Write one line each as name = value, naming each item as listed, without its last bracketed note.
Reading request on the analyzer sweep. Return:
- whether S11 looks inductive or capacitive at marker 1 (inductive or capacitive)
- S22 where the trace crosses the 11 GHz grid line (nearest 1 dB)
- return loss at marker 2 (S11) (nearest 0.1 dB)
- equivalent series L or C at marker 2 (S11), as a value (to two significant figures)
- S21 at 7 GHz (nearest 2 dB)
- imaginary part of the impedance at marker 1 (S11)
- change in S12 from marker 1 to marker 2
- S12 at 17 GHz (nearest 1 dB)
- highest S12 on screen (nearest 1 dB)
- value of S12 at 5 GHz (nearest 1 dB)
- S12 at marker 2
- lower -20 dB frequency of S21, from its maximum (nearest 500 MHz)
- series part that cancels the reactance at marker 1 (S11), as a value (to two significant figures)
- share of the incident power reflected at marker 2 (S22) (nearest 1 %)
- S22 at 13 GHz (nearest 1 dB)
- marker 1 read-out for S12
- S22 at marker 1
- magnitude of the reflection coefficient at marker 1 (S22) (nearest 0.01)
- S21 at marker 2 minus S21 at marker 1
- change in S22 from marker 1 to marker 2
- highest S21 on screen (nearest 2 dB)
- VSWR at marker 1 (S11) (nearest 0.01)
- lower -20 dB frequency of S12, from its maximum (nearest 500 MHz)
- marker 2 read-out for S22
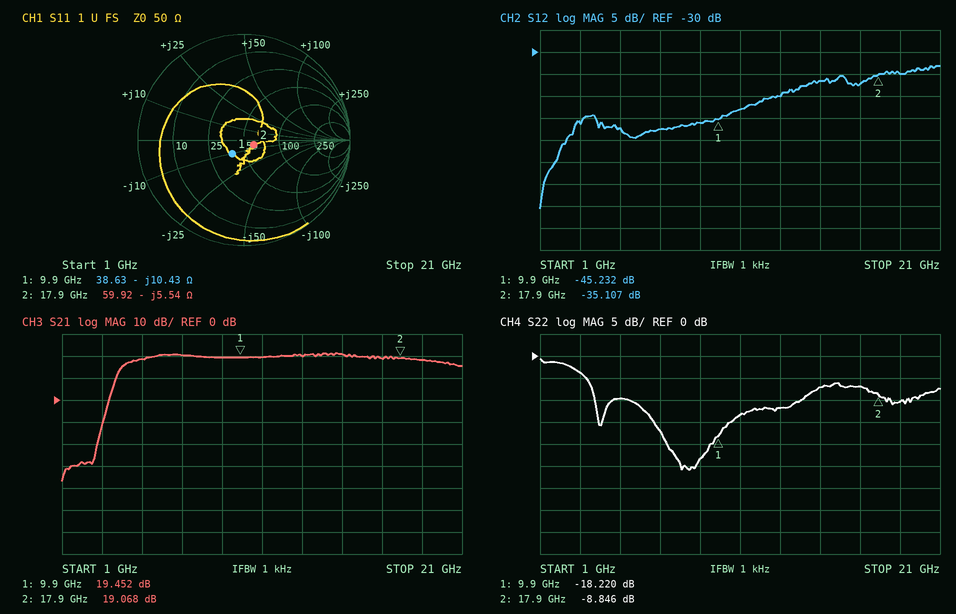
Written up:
whether S11 looks inductive or capacitive at marker 1 = capacitive
S22 where the trace crosses the 11 GHz grid line = -13 dB
return loss at marker 2 (S11) = 19.7 dB
equivalent series L or C at marker 2 (S11), as a value = 1.6 pF
S21 at 7 GHz = 20 dB
imaginary part of the impedance at marker 1 = -10.43 Ω
change in S12 from marker 1 to marker 2 = 10.125 dB
S12 at 17 GHz = -37 dB
highest S12 on screen = -33 dB
value of S12 at 5 GHz = -47 dB
S12 at marker 2 = -35.107 dB
lower -20 dB frequency of S21, from its maximum = 3.5 GHz
series part that cancels the reactance at marker 1 (S11), as a value = 170 pH
share of the incident power reflected at marker 2 (S22) = 13 %
S22 at 13 GHz = -12 dB
marker 1 read-out for S12 = -45.232 dB
S22 at marker 1 = -18.220 dB
magnitude of the reflection coefficient at marker 1 (S22) = 0.12
S21 at marker 2 minus S21 at marker 1 = -0.384 dB
change in S22 from marker 1 to marker 2 = 9.374 dB
highest S21 on screen = 22 dB
VSWR at marker 1 (S11) = 1.42
lower -20 dB frequency of S12, from its maximum = 2.0 GHz
marker 2 read-out for S22 = -8.846 dB
